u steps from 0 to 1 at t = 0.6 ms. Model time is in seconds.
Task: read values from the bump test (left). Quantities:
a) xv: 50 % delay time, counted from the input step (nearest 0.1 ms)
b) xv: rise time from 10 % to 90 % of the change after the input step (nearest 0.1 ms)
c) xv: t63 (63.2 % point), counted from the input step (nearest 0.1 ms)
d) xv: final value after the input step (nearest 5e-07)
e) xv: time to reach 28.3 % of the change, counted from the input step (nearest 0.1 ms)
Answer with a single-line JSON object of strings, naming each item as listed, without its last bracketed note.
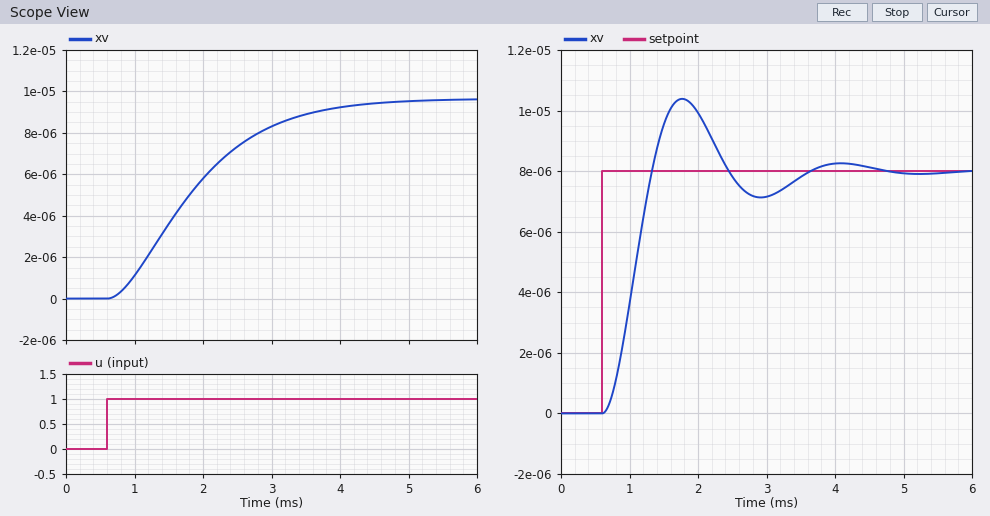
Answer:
{"xv: 50 % delay time, counted from the input step": "1.2 ms", "xv: rise time from 10 % to 90 % of the change after the input step": "2.3 ms", "xv: t63 (63.2 % point), counted from the input step": "1.5 ms", "xv: final value after the input step": "0.0000095", "xv: time to reach 28.3 % of the change, counted from the input step": "0.7 ms"}
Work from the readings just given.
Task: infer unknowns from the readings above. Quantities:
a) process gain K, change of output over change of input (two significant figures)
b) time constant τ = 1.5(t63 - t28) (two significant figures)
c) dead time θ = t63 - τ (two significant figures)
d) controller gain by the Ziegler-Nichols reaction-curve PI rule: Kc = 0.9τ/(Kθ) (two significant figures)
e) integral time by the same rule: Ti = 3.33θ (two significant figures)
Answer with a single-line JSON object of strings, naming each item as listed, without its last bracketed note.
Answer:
{"process gain K, change of output over change of input": "0.0000095", "time constant τ = 1.5(t63 - t28)": "1.2 ms", "dead time θ = t63 - τ": "0.30 ms", "controller gain by the Ziegler-Nichols reaction-curve PI rule: Kc = 0.9τ/(Kθ)": "380000", "integral time by the same rule: Ti = 3.33θ": "1.00 ms"}
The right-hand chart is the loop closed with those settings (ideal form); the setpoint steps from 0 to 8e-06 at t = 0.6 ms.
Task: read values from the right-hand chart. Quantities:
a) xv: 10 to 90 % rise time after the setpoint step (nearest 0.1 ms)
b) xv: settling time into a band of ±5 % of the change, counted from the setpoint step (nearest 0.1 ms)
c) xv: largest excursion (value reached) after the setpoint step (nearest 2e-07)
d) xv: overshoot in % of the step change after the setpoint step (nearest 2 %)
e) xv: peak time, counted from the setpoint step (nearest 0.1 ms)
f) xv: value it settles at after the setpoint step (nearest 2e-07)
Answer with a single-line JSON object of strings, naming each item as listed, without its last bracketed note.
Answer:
{"xv: 10 to 90 % rise time after the setpoint step": "0.5 ms", "xv: settling time into a band of ±5 % of the change, counted from the setpoint step": "2.8 ms", "xv: largest excursion (value reached) after the setpoint step": "0.0000104", "xv: overshoot in % of the step change after the setpoint step": "30 %", "xv: peak time, counted from the setpoint step": "1.2 ms", "xv: value it settles at after the setpoint step": "0.0000080"}
